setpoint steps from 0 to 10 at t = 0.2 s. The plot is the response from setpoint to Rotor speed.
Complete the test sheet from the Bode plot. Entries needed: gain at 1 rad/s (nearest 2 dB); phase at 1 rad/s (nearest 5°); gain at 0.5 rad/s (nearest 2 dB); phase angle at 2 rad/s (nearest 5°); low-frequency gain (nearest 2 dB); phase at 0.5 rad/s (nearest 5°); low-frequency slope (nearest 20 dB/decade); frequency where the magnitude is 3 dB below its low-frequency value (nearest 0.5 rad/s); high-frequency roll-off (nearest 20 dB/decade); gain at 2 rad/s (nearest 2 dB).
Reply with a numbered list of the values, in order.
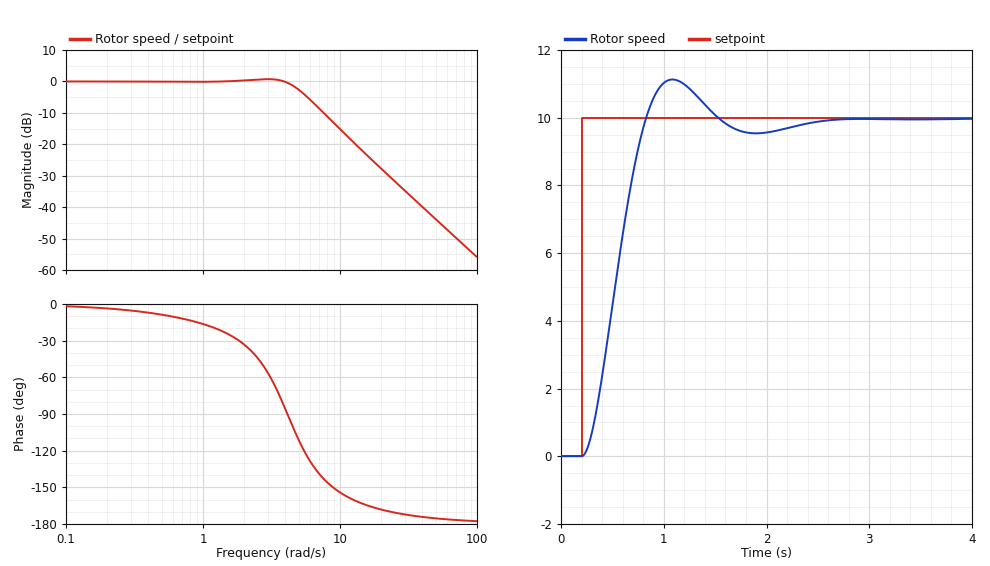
1. 0 dB
2. -15°
3. 0 dB
4. -35°
5. 0 dB
6. -10°
7. 0 dB/decade
8. 5.0 rad/s
9. -40 dB/decade
10. 0 dB
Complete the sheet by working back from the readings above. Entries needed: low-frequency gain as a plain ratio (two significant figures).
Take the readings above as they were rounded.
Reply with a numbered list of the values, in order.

1. 1.0
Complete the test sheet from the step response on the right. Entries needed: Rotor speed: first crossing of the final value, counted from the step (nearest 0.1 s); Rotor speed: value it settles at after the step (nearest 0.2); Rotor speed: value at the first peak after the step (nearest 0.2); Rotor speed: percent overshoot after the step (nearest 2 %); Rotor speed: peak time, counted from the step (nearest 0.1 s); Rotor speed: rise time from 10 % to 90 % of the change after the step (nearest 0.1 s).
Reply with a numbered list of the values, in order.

1. 0.6 s
2. 10.0
3. 11.2
4. 12 %
5. 0.9 s
6. 0.4 s
